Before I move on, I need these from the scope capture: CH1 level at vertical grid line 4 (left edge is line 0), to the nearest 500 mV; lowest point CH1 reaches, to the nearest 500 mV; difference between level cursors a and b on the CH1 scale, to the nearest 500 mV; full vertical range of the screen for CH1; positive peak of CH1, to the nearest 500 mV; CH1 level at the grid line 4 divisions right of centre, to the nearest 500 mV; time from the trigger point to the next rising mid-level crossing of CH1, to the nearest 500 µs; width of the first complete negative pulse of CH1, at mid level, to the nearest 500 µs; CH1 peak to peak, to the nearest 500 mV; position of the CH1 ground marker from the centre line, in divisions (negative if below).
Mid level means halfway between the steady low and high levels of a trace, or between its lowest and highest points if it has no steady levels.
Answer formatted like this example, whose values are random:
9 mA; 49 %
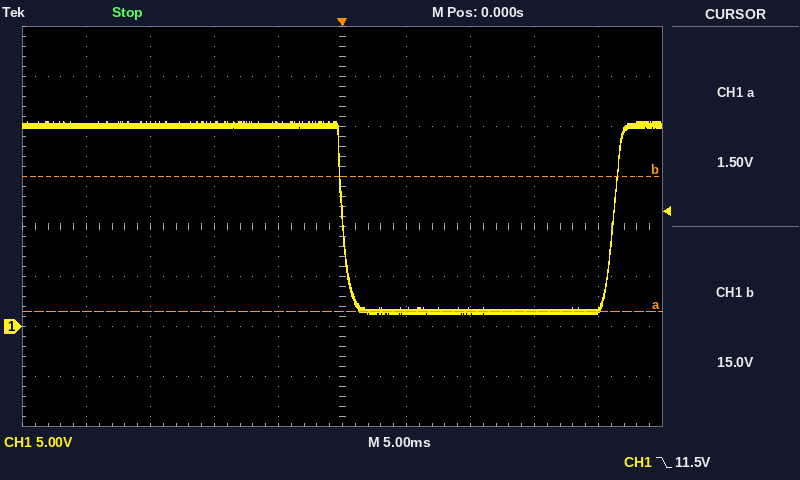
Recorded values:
20.0 V; 1.5 V; 13.5 V; 40 V; 20.5 V; 2.0 V; 21.0 ms; 21.0 ms; 19.0 V; -2.0 div
